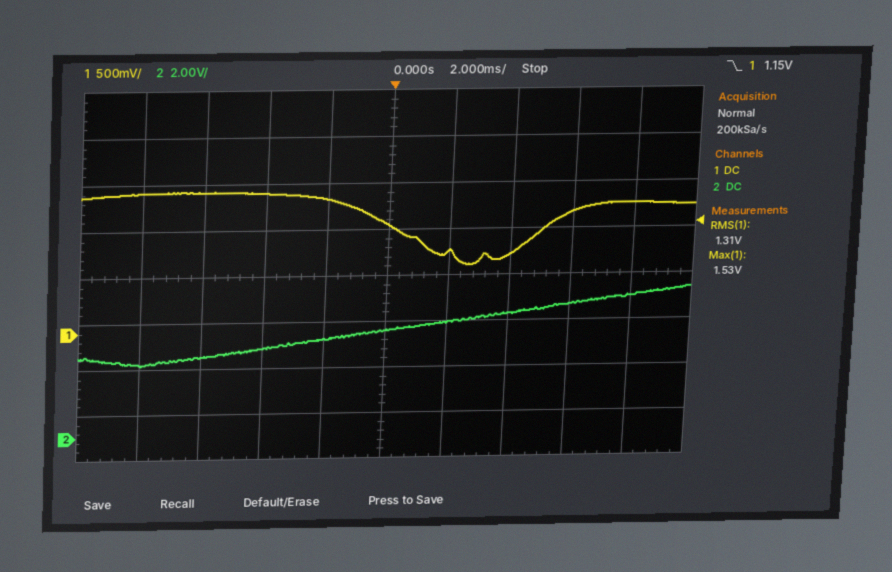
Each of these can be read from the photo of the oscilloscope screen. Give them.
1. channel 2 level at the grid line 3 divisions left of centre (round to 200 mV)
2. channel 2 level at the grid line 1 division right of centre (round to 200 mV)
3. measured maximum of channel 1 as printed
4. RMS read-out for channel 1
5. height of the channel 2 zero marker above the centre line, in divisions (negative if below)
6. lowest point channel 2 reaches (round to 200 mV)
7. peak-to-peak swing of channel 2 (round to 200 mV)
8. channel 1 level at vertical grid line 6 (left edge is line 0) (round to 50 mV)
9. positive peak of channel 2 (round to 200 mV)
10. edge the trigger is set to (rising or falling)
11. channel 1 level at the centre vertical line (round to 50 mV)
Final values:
3.6 V
5.0 V
1.53 V
1.31 V
-3.5 div
3.2 V
3.2 V
850 mV
6.4 V
falling
1.15 V
